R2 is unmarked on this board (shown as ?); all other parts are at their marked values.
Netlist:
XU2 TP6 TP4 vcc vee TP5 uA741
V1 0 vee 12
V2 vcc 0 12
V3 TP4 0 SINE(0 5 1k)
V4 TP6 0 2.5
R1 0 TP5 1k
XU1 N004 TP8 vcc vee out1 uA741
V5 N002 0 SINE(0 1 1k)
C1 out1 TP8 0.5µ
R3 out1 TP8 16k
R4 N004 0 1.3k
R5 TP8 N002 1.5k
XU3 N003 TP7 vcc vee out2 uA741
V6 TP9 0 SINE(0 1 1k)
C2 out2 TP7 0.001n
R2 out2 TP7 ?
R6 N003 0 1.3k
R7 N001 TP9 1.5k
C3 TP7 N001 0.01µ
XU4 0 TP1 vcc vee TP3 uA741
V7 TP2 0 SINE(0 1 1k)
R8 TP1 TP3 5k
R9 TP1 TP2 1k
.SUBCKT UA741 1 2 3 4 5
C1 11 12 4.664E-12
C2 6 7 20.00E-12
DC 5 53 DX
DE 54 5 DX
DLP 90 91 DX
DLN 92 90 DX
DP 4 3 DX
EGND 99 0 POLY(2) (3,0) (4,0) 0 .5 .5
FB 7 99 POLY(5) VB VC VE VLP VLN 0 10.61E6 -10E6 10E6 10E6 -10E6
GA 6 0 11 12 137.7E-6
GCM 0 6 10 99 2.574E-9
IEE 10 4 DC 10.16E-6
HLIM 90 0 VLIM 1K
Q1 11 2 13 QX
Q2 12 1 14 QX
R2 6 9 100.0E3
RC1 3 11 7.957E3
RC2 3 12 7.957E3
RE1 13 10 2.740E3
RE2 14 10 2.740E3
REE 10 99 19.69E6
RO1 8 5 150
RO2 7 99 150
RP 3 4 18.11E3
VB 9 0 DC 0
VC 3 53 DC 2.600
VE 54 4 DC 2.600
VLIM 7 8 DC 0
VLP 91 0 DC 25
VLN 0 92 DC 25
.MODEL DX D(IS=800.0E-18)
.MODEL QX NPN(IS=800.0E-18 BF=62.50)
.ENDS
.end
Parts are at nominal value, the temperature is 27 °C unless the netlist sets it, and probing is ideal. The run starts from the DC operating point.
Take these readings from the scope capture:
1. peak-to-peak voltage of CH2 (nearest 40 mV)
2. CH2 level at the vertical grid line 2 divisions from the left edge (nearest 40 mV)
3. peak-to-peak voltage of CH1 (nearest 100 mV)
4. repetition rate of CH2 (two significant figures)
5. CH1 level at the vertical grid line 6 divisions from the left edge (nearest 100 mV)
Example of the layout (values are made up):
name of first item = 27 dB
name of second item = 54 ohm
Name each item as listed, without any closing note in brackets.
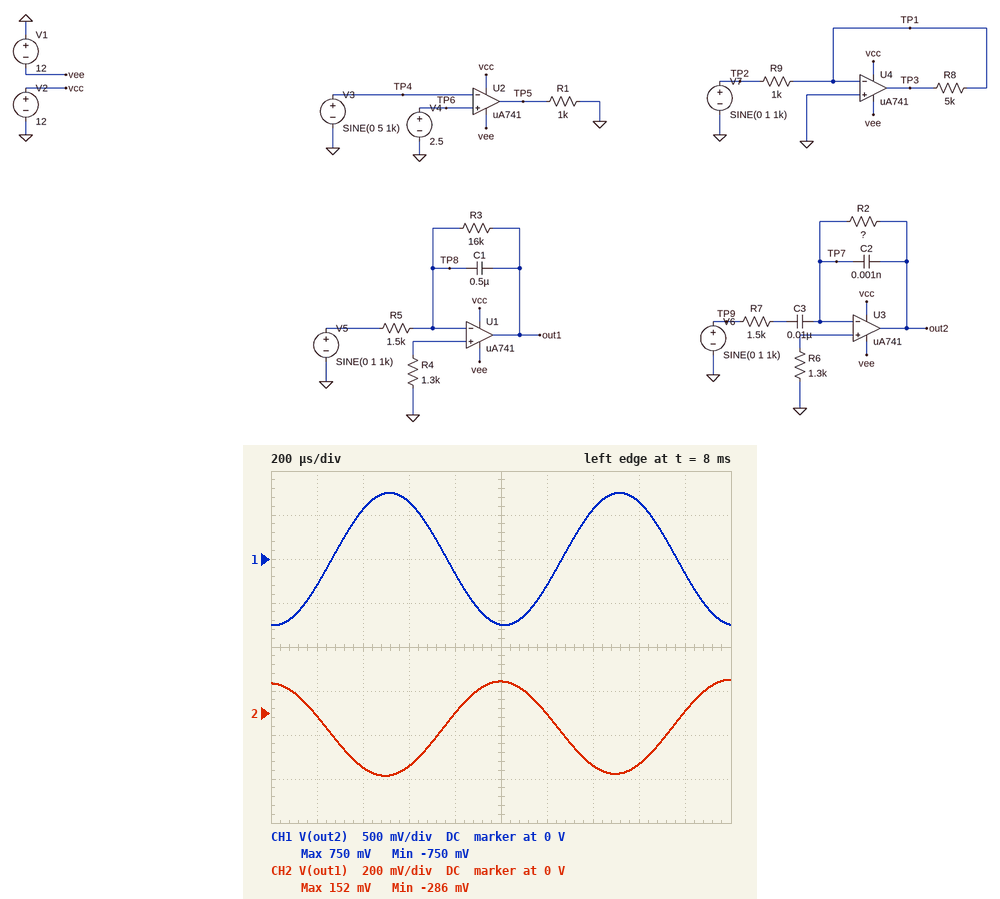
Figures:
peak-to-peak voltage of CH2 = 440 mV
CH2 level at the vertical grid line 2 divisions from the left edge = -240 mV
peak-to-peak voltage of CH1 = 1.5 V
repetition rate of CH2 = 1.0 kHz
CH1 level at the vertical grid line 6 divisions from the left edge = -300 mV
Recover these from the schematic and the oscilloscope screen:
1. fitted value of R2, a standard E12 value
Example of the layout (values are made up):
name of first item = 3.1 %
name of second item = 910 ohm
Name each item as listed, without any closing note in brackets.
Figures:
fitted value of R2, a standard E12 value = 12 kΩ
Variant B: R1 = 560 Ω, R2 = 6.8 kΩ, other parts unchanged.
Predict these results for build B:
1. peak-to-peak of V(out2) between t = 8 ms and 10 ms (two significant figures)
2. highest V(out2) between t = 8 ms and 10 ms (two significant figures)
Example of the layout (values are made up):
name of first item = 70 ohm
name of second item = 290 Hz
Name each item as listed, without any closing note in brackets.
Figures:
peak-to-peak of V(out2) between t = 8 ms and 10 ms = 850 mV
highest V(out2) between t = 8 ms and 10 ms = 430 mV
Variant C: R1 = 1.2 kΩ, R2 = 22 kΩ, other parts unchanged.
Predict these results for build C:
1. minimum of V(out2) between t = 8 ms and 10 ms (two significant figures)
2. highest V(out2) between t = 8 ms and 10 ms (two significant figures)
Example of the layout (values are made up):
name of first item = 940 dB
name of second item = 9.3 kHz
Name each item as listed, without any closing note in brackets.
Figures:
minimum of V(out2) between t = 8 ms and 10 ms = -1.4 V
highest V(out2) between t = 8 ms and 10 ms = 1.4 V
